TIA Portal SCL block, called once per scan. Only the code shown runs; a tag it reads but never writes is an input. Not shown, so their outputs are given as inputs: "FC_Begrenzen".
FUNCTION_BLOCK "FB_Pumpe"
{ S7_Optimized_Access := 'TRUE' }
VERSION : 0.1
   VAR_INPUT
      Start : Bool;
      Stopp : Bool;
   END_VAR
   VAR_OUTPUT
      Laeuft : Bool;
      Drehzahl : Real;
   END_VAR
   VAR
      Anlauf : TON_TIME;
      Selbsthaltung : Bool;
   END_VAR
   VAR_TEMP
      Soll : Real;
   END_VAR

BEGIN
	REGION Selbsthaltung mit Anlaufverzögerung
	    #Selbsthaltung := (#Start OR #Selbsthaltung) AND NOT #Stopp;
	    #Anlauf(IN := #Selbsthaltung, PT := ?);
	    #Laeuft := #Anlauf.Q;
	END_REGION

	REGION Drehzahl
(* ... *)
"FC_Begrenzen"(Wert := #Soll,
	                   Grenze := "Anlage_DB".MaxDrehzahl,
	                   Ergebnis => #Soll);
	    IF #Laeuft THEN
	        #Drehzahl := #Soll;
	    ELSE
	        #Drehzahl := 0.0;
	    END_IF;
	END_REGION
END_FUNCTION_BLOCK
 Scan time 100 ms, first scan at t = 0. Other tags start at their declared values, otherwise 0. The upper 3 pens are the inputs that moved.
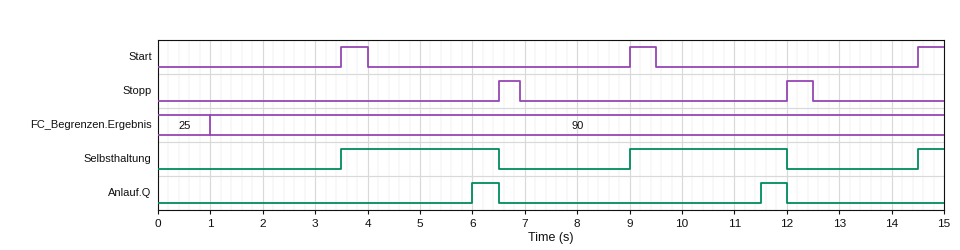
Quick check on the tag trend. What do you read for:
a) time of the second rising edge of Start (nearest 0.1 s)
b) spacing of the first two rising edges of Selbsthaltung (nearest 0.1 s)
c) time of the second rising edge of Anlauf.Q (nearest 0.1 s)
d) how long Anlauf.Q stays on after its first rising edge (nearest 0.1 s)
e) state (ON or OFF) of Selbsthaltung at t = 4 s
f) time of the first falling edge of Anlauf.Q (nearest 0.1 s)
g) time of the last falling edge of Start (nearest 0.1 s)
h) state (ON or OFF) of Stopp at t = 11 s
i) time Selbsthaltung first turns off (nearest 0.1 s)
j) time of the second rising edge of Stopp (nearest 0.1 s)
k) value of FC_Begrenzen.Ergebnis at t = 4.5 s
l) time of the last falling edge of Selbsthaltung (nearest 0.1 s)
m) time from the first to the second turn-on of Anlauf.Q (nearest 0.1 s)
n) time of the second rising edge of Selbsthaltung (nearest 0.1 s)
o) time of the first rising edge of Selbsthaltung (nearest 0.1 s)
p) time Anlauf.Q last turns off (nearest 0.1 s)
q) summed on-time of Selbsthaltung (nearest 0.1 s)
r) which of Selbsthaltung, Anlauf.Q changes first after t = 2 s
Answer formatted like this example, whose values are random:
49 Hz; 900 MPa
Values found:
9.0 s; 5.5 s; 11.5 s; 0.5 s; ON; 6.5 s; 9.5 s; OFF; 6.5 s; 12.0 s; 90; 12.0 s; 5.5 s; 9.0 s; 3.5 s; 12.0 s; 6.5 s; Selbsthaltung
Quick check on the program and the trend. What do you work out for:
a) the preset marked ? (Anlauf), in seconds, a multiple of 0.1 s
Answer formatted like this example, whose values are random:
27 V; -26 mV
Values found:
2.5 s
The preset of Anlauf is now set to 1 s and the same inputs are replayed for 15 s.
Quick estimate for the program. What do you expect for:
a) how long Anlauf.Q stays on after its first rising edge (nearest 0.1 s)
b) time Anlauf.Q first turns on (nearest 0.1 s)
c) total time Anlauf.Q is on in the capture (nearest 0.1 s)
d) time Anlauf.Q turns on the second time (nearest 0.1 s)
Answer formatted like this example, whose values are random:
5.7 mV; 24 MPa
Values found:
2.0 s; 4.5 s; 4.0 s; 10.0 s
